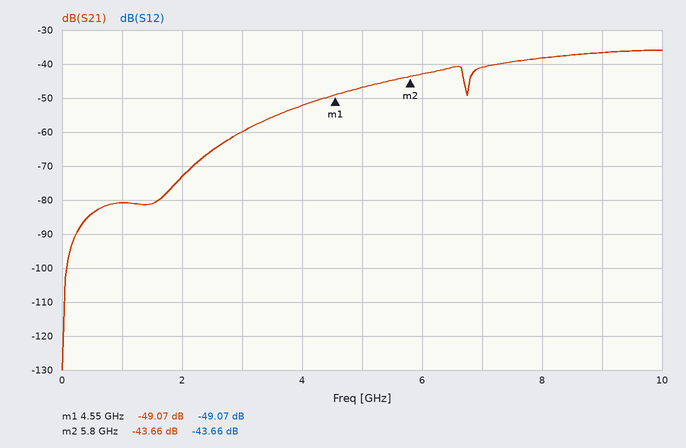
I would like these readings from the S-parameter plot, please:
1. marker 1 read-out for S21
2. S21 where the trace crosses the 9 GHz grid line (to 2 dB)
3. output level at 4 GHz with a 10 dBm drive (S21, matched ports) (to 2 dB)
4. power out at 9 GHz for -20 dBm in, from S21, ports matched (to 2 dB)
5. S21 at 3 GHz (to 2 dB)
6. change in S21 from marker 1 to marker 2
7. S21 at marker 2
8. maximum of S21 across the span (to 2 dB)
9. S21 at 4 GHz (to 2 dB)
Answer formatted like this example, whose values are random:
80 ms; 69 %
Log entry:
-49.07 dB; -36 dB; -42 dBm; -56 dBm; -60 dB; 5.41 dB; -43.66 dB; -36 dB; -52 dB
